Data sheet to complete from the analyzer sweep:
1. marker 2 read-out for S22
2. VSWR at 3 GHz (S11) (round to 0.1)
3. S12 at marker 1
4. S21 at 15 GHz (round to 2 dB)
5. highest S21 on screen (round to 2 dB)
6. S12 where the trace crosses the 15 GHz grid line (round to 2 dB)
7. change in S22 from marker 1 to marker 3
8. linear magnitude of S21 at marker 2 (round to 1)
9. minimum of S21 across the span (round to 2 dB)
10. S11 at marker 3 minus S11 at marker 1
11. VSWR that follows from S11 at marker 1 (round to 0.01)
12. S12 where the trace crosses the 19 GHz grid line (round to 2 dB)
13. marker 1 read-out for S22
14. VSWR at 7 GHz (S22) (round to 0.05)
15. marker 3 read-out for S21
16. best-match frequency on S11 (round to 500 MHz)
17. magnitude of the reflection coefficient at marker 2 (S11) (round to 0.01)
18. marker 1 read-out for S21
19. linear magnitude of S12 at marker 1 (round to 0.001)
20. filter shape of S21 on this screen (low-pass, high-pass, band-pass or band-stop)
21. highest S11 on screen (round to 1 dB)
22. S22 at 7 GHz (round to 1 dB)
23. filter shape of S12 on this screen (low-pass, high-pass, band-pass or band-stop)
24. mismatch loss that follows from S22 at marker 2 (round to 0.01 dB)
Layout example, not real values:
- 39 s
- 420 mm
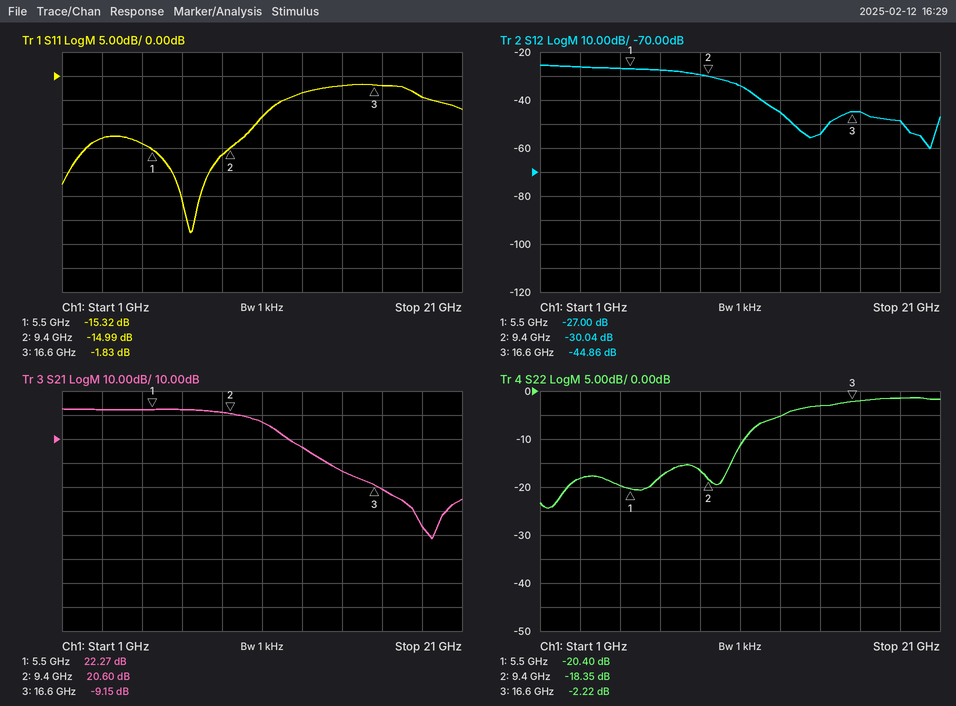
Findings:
- -18.35 dB
- 1.6
- -27.00 dB
- -4 dB
- 22 dB
- -54 dB
- 18.18 dB
- 11
- -32 dB
- 13.49 dB
- 1.41
- -48 dB
- -20.40 dB
- 1.30
- -9.15 dB
- 7.5 GHz
- 0.18
- 22.27 dB
- 0.045
- low-pass
- -2 dB
- -18 dB
- low-pass
- 0.06 dB
